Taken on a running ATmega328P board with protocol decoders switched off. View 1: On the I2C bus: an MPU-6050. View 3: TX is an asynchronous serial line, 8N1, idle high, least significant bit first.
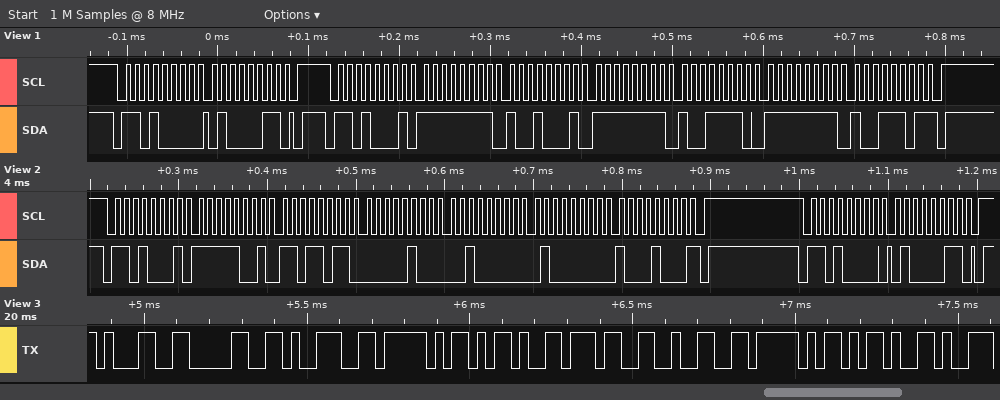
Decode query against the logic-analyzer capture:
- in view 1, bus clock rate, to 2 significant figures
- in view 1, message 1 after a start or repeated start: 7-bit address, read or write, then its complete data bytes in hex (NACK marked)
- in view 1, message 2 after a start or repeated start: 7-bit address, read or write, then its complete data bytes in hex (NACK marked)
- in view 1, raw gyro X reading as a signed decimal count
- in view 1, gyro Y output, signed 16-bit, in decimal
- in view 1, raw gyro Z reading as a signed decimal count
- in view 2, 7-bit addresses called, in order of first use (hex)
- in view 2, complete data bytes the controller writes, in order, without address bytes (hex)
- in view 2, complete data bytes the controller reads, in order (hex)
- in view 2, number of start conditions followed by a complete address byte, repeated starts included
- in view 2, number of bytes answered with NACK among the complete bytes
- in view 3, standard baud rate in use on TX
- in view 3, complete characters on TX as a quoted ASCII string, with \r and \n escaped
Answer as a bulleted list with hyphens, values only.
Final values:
- 100 kHz
- 0x68 write: 43
- 0x68 read: FF 91 FF 9E FF 9D NACK
- -111
- -98
- -99
- 0x68
- 43
- F9 DB 04 20 40 88
- 2
- 1
- 38400 baud
- "109_-72_-"
